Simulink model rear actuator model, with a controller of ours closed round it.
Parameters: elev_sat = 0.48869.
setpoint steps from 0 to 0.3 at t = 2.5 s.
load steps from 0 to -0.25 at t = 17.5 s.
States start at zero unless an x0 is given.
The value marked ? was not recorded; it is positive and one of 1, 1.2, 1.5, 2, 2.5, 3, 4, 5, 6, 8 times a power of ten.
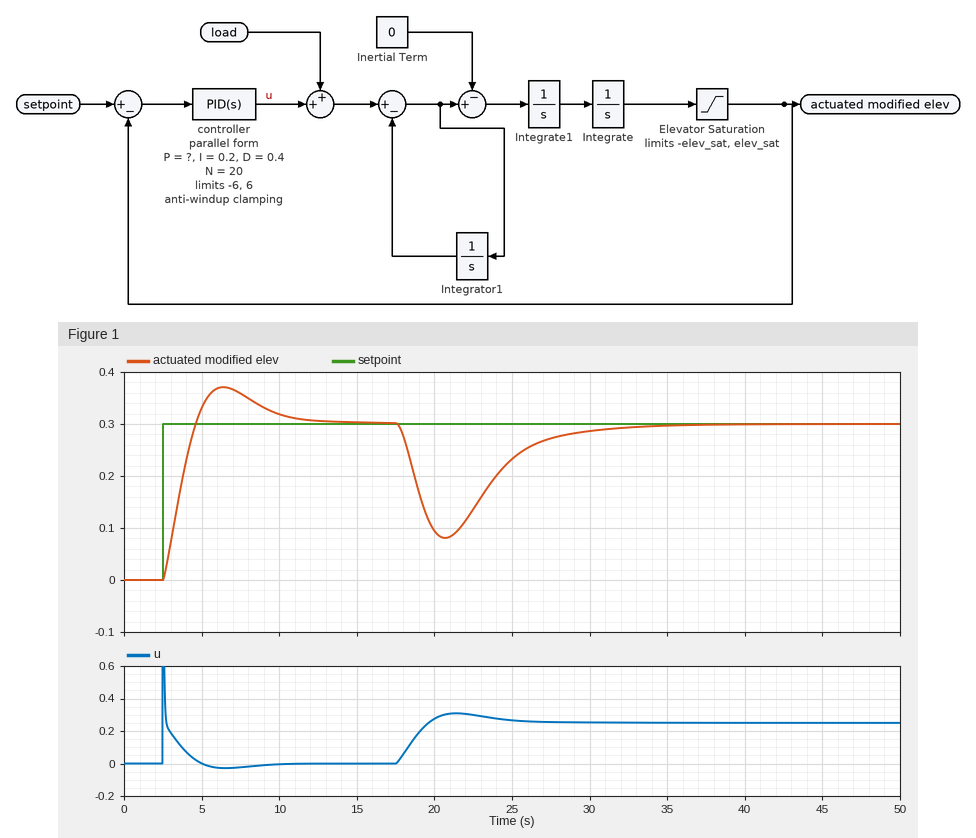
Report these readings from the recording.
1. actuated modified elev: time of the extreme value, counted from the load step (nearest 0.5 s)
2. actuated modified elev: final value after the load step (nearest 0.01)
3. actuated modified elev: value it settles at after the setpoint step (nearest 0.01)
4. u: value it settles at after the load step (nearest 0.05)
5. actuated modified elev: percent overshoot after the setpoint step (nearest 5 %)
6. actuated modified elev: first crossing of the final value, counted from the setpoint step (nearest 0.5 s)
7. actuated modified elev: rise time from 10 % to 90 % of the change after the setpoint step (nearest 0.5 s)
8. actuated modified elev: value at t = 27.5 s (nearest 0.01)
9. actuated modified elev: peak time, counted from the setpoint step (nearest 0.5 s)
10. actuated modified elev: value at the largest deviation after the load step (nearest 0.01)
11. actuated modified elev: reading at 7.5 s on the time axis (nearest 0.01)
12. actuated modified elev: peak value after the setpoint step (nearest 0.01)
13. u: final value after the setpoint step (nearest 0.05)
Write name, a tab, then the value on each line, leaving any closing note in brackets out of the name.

actuated modified elev: time of the extreme value, counted from the load step	3.0 s
actuated modified elev: final value after the load step	0.30
actuated modified elev: value it settles at after the setpoint step	0.30
u: value it settles at after the load step	0.25
actuated modified elev: percent overshoot after the setpoint step	25 %
actuated modified elev: first crossing of the final value, counted from the setpoint step	2.0 s
actuated modified elev: rise time from 10 % to 90 % of the change after the setpoint step	1.5 s
actuated modified elev: value at t = 27.5 s	0.27
actuated modified elev: peak time, counted from the setpoint step	4.0 s
actuated modified elev: value at the largest deviation after the load step	0.08
actuated modified elev: reading at 7.5 s on the time axis	0.36
actuated modified elev: peak value after the setpoint step	0.37
u: final value after the setpoint step	0.00
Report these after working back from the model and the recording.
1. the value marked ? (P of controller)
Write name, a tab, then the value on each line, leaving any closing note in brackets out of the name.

the value marked ?	1
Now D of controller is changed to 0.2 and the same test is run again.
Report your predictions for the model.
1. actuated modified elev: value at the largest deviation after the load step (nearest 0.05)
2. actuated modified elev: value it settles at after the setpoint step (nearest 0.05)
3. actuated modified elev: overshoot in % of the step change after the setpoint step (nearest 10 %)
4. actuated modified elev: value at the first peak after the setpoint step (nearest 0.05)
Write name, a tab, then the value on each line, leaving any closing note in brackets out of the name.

actuated modified elev: value at the largest deviation after the load step	0.05
actuated modified elev: value it settles at after the setpoint step	0.30
actuated modified elev: overshoot in % of the step change after the setpoint step	30 %
actuated modified elev: value at the first peak after the setpoint step	0.40
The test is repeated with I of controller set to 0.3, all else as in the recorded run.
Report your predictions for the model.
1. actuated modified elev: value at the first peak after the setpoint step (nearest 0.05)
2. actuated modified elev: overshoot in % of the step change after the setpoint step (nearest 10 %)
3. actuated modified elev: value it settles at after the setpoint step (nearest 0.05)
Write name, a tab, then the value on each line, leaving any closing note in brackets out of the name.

actuated modified elev: value at the first peak after the setpoint step	0.40
actuated modified elev: overshoot in % of the step change after the setpoint step	30 %
actuated modified elev: value it settles at after the setpoint step	0.30
